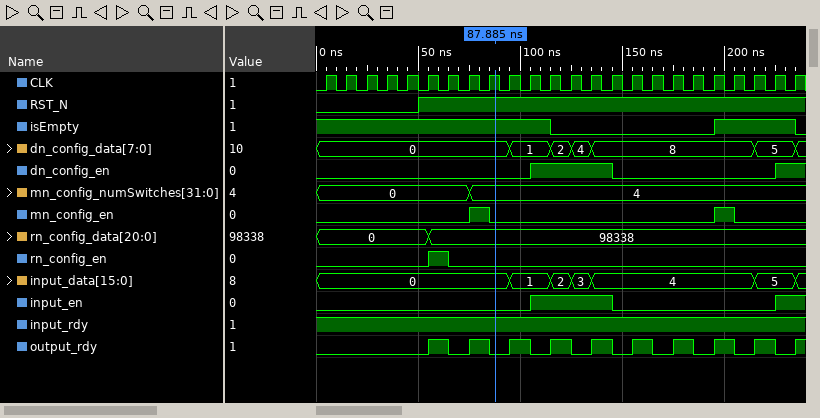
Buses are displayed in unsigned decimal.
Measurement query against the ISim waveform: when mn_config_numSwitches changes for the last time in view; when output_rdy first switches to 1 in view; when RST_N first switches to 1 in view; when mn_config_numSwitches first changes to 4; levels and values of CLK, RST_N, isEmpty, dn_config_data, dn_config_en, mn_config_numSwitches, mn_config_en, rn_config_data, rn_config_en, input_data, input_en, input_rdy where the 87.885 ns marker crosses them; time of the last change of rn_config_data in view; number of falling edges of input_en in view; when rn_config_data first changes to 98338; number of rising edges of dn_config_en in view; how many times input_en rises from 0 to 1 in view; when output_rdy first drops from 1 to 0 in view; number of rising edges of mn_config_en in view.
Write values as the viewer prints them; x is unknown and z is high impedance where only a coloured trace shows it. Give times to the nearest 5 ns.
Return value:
75 ns
55 ns
50 ns
75 ns
CLK=1, RST_N=1, isEmpty=1, dn_config_data=0, dn_config_en=0, mn_config_numSwitches=4, mn_config_en=0, rn_config_data=98338, rn_config_en=0, input_data=0, input_en=0, input_rdy=1
55 ns
1
55 ns
2
2
65 ns
2
